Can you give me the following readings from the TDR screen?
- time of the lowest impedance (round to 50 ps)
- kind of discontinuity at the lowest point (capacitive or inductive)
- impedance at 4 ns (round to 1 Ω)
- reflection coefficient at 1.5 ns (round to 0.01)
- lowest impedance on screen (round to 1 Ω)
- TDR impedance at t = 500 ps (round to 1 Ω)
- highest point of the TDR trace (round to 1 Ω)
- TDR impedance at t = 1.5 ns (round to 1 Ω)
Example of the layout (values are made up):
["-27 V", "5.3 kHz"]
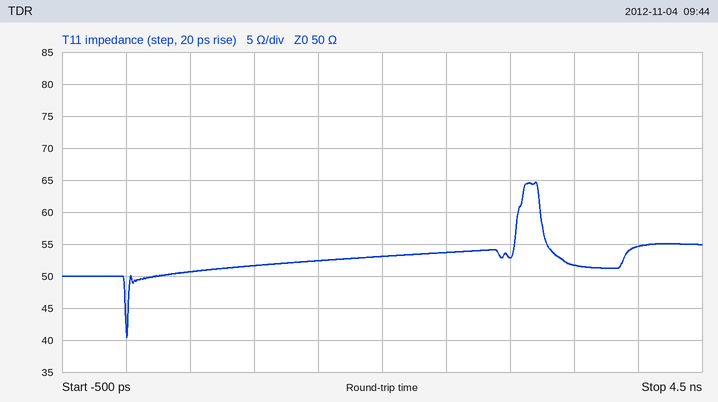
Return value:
["0 ps", "capacitive", "55 Ω", "+0.02", "40 Ω", "51 Ω", "65 Ω", "52 Ω"]
